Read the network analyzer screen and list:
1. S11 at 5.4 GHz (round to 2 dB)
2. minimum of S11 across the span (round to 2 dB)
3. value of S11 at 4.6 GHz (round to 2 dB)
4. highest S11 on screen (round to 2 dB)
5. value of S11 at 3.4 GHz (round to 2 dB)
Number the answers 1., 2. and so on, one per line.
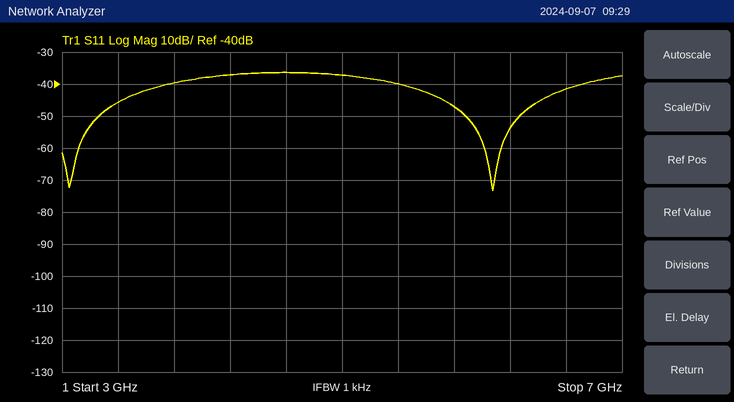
1. -40 dB
2. -74 dB
3. -36 dB
4. -36 dB
5. -46 dB
